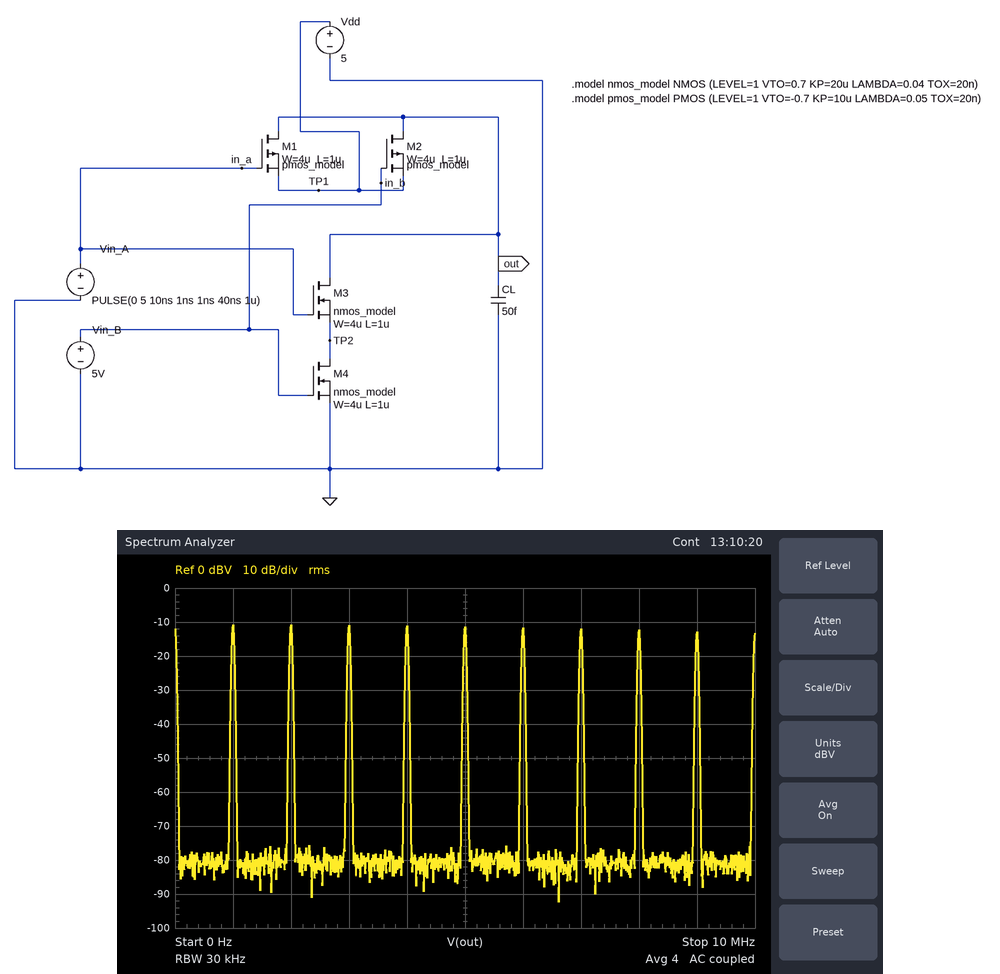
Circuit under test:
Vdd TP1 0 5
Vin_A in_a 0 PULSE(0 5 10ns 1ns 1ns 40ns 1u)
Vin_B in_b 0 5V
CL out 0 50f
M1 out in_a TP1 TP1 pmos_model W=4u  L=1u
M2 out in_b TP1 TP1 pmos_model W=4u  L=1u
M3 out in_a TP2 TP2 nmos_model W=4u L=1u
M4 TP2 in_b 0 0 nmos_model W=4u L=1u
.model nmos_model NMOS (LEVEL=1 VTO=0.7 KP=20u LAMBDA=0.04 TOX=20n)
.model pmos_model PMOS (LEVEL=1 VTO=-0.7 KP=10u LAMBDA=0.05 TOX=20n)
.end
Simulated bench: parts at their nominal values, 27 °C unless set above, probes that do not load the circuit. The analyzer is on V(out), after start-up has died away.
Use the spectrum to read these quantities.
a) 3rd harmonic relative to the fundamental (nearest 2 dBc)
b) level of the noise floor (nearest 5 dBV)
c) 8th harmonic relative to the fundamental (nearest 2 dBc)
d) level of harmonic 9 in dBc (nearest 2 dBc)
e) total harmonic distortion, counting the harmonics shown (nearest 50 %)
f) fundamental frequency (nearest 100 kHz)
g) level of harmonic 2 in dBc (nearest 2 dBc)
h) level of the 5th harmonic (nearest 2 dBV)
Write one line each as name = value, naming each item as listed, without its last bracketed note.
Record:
3rd harmonic relative to the fundamental = 0 dBc
level of the noise floor = -80 dBV
8th harmonic relative to the fundamental = -2 dBc
level of harmonic 9 in dBc = -2 dBc
total harmonic distortion, counting the harmonics shown = 250 %
fundamental frequency = 1.0 MHz
level of harmonic 2 in dBc = 0 dBc
level of the 5th harmonic = -12 dBV
